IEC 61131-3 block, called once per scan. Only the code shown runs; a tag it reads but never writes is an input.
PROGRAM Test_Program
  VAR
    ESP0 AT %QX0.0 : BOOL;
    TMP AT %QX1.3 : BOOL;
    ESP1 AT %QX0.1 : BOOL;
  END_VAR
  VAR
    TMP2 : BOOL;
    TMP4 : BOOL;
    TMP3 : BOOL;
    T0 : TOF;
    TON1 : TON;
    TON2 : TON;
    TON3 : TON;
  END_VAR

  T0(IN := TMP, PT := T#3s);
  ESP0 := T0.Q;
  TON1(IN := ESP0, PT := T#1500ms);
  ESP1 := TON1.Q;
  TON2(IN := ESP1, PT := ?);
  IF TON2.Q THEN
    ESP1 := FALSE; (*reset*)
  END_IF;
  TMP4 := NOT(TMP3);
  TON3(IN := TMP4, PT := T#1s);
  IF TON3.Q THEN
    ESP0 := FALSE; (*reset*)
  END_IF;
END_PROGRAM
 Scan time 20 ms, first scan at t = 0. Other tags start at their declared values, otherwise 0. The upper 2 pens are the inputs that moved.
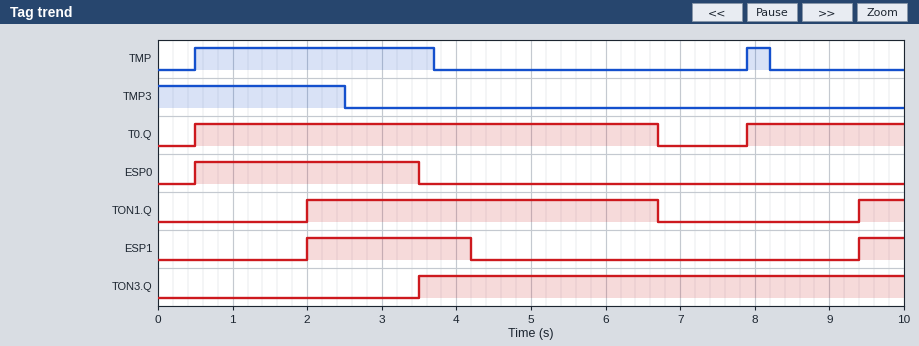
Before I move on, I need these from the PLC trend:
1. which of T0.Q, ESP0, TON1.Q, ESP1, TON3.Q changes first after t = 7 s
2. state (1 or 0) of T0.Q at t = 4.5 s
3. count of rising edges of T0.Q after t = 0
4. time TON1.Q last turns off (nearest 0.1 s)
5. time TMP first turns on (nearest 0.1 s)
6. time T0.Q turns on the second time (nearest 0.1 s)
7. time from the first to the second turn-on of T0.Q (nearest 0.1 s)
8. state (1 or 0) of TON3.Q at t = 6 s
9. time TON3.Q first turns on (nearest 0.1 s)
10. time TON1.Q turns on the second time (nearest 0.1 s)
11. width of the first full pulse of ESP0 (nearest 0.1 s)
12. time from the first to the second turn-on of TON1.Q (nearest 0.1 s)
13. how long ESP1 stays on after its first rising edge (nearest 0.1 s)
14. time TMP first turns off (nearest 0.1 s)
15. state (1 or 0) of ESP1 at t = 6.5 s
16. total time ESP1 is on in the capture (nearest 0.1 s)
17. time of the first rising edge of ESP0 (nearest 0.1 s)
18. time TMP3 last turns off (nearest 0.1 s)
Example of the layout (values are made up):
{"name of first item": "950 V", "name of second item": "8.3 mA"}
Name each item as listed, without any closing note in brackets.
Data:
{"which of T0.Q, ESP0, TON1.Q, ESP1, TON3.Q changes first after t = 7 s": "T0.Q", "state (1 or 0) of T0.Q at t = 4.5 s": "1", "count of rising edges of T0.Q after t = 0": "2", "time TON1.Q last turns off": "6.7 s", "time TMP first turns on": "0.5 s", "time T0.Q turns on the second time": "7.9 s", "time from the first to the second turn-on of T0.Q": "7.4 s", "state (1 or 0) of TON3.Q at t = 6 s": "1", "time TON3.Q first turns on": "3.5 s", "time TON1.Q turns on the second time": "9.4 s", "width of the first full pulse of ESP0": "3.0 s", "time from the first to the second turn-on of TON1.Q": "7.4 s", "how long ESP1 stays on after its first rising edge": "2.2 s", "time TMP first turns off": "3.7 s", "state (1 or 0) of ESP1 at t = 6.5 s": "0", "total time ESP1 is on in the capture": "2.8 s", "time of the first rising edge of ESP0": "0.5 s", "time TMP3 last turns off": "2.5 s"}
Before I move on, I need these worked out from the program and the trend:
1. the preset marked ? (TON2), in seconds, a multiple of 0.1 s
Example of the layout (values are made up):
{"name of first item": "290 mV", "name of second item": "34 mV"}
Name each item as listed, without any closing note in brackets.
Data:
{"the preset marked ? (TON2), in seconds, a multiple of 0.1 s": "2.2 s"}
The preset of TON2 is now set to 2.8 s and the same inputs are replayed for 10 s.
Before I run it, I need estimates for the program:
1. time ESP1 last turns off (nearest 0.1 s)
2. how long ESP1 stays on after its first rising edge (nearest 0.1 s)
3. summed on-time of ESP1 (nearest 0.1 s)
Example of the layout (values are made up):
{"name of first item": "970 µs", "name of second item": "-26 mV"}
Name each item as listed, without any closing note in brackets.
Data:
{"time ESP1 last turns off": "4.8 s", "how long ESP1 stays on after its first rising edge": "2.8 s", "summed on-time of ESP1": "3.4 s"}
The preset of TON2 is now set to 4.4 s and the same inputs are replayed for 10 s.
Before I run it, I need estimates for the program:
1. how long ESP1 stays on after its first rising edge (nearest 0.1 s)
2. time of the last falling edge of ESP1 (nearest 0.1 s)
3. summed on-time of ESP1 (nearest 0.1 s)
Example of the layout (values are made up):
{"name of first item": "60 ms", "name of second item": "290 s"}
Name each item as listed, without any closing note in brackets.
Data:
{"how long ESP1 stays on after its first rising edge": "4.4 s", "time of the last falling edge of ESP1": "6.4 s", "summed on-time of ESP1": "5.0 s"}
